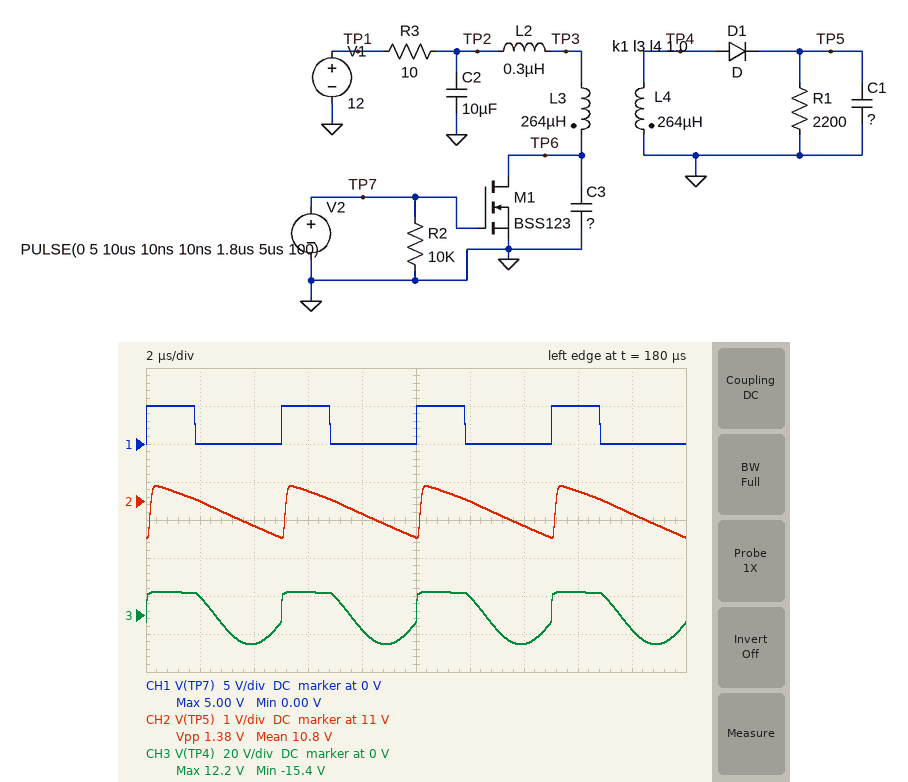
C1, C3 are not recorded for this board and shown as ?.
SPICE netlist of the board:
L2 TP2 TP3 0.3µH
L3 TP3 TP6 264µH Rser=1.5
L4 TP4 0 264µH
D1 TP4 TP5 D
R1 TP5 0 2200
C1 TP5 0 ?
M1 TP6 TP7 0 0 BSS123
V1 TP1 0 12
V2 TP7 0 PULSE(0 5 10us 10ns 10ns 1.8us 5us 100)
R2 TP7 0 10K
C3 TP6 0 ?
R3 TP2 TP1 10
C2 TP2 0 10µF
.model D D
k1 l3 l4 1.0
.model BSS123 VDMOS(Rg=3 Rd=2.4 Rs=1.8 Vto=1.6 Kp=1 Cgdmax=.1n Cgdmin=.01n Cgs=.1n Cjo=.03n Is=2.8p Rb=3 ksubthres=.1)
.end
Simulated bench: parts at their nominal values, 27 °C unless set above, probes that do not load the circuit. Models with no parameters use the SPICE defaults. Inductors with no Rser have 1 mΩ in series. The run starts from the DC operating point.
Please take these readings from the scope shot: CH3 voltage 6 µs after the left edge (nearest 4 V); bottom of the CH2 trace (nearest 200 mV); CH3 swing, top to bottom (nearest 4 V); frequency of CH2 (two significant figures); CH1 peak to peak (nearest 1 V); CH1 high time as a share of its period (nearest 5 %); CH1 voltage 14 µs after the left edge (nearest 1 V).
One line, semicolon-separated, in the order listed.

12 V; 10.0 V; 28 V; 200 kHz; 5 V; 35 %; 0 V
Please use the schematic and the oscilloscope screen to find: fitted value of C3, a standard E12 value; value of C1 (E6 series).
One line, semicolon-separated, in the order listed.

2.7 nF; 15 nF
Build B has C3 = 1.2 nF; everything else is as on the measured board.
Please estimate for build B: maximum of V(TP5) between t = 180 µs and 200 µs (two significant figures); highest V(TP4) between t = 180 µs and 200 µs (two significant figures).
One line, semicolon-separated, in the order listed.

12 V; 13 V
